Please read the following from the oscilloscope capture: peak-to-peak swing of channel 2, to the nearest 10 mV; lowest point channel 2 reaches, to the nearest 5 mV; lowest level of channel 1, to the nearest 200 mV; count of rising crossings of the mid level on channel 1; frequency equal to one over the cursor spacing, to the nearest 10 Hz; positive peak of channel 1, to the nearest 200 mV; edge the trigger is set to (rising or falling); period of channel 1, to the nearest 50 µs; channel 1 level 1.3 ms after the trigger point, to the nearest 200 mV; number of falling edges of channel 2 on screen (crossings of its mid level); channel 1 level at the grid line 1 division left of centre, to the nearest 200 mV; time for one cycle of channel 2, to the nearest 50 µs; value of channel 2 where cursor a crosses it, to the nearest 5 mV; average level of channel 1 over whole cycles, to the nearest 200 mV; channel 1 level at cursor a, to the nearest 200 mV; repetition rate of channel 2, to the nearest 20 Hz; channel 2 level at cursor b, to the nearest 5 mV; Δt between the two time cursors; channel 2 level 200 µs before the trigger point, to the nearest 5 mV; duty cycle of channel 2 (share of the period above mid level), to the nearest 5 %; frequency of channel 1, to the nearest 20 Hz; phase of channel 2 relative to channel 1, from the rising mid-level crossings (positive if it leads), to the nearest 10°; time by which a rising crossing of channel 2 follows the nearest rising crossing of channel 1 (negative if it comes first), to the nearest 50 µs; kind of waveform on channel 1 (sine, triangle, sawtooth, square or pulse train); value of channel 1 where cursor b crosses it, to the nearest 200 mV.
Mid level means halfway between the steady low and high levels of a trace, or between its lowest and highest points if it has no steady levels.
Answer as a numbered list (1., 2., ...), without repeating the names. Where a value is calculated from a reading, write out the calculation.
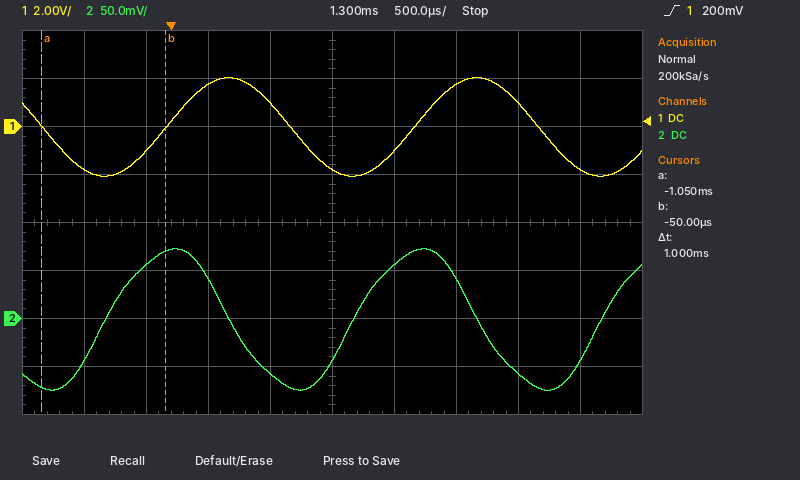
1. 150 mV
2. -75 mV
3. -2.0 V
4. 2
5. 1 / 1 ms ≈ 1.00 kHz
6. 2.0 V
7. rising
8. 2.00 ms
9. -1.8 V
10. 2
11. 1.0 V
12. 2.00 ms
13. -70 mV
14. (2.0 V + (-2.0 V)) / 2 ≈ 0.0 V
15. 0.0 V
16. 1 / 2.00 ms ≈ 500 Hz
17. 70 mV
18. 1 ms
19. 55 mV
20. 50 %
21. 1 / 2.00 ms ≈ 500 Hz
22. −360° × (-500 µs) / 2.00 ms ≈ +90°
23. -500 µs
24. sine
25. 0.0 V
